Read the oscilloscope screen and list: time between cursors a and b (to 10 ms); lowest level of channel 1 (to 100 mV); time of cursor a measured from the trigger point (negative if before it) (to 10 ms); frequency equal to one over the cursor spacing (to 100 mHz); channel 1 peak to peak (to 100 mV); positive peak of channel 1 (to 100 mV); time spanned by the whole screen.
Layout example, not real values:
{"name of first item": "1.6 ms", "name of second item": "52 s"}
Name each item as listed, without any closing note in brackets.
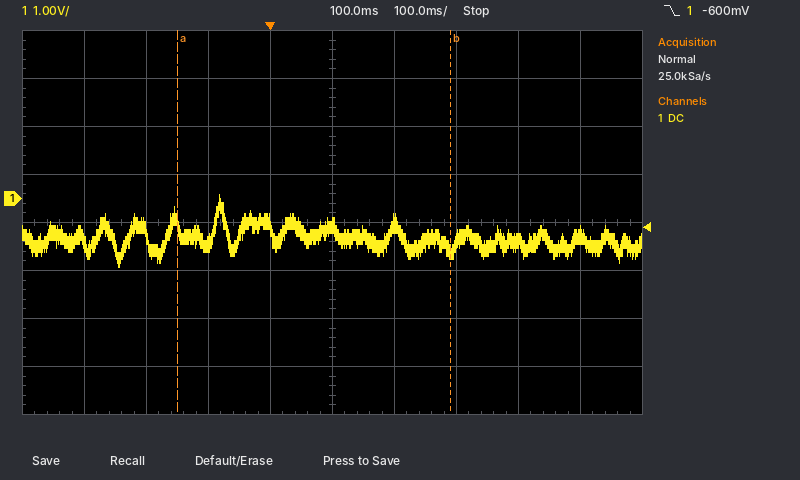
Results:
{"time between cursors a and b": "440 ms", "lowest level of channel 1": "-1.4 V", "time of cursor a measured from the trigger point (negative if before it)": "-150 ms", "frequency equal to one over the cursor spacing": "2.3 Hz", "channel 1 peak to peak": "1.5 V", "positive peak of channel 1": "100 mV", "time spanned by the whole screen": "1 s"}
